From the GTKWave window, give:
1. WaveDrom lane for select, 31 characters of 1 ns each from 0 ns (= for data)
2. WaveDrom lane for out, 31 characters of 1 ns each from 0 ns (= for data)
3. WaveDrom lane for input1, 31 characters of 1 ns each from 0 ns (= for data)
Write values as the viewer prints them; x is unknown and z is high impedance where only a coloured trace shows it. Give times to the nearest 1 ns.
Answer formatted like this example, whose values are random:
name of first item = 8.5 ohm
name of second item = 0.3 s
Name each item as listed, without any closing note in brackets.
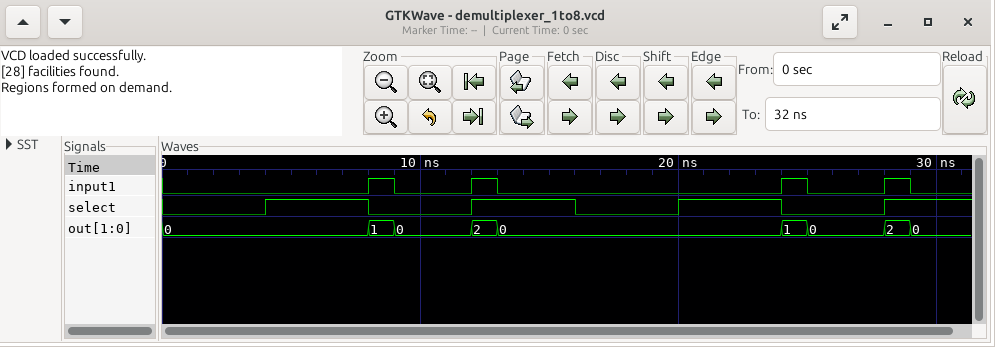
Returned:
WaveDrom lane for select, 31 characters of 1 ns each from 0 ns = {name: 'select', wave: '0...1...0...1...0...1...0...1..'}
WaveDrom lane for out, 31 characters of 1 ns each from 0 ns = {name: 'out', wave: '=.......==..==..........==..==.', data: '0 1 0 2 0 1 0 2 0'}
WaveDrom lane for input1, 31 characters of 1 ns each from 0 ns = {name: 'input1', wave: '0.......10..10..........10..10.'}
